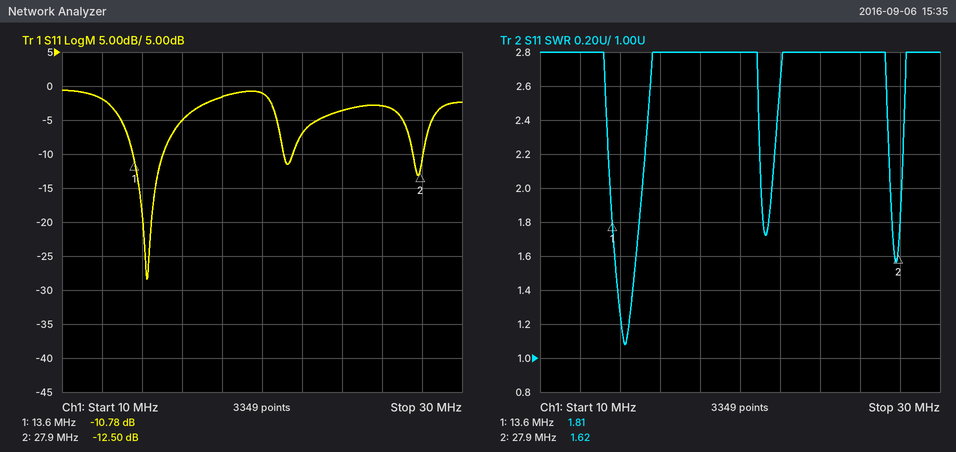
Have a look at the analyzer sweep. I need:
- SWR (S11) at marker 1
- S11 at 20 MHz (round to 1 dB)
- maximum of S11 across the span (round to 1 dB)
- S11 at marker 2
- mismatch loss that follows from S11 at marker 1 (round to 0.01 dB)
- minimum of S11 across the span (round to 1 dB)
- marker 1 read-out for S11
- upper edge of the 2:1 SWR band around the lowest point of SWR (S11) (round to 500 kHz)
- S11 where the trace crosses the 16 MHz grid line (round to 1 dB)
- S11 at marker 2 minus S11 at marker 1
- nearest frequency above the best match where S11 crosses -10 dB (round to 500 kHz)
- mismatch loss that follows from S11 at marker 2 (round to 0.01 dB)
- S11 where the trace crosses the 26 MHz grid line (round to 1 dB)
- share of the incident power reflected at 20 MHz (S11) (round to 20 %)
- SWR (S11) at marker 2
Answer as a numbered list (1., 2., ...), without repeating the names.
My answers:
1. 1.81
2. -1 dB
3. -1 dB
4. -12.50 dB
5. 0.38 dB
6. -28 dB
7. -10.78 dB
8. 15.0 MHz
9. -5 dB
10. -1.72 dB
11. 15.0 MHz
12. 0.25 dB
13. -3 dB
14. 80 %
15. 1.62
